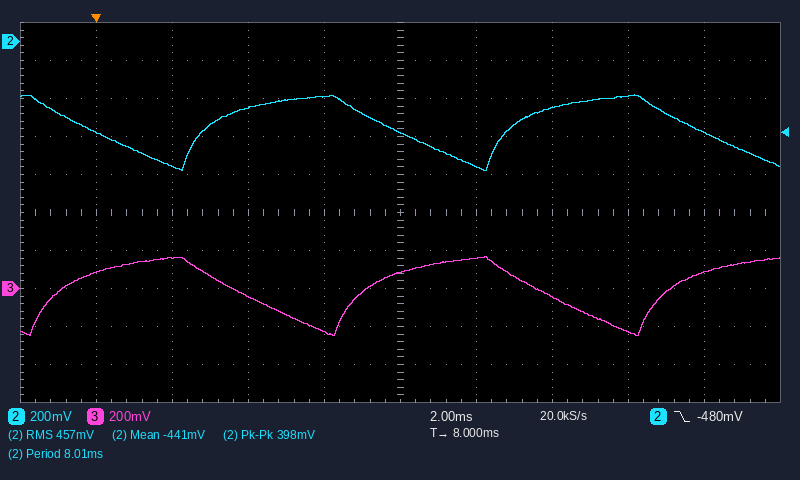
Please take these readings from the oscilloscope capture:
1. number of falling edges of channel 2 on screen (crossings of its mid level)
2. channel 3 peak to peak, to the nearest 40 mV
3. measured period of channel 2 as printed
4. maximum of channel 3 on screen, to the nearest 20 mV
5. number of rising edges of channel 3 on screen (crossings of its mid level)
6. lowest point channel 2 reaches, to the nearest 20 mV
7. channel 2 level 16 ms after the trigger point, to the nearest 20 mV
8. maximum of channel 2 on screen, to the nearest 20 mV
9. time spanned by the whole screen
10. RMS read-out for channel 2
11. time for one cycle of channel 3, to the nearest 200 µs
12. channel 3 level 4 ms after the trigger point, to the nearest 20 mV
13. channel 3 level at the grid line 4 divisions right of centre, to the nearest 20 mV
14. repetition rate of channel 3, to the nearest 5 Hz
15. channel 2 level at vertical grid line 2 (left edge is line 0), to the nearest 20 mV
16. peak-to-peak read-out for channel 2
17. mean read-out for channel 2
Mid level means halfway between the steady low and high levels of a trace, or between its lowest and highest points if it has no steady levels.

3
400 mV
8.01 ms
160 mV
3
-680 mV
-480 mV
-280 mV
20 ms
457 mV
8.0 ms
-40 mV
80 mV
125 Hz
-660 mV
398 mV
-441 mV
